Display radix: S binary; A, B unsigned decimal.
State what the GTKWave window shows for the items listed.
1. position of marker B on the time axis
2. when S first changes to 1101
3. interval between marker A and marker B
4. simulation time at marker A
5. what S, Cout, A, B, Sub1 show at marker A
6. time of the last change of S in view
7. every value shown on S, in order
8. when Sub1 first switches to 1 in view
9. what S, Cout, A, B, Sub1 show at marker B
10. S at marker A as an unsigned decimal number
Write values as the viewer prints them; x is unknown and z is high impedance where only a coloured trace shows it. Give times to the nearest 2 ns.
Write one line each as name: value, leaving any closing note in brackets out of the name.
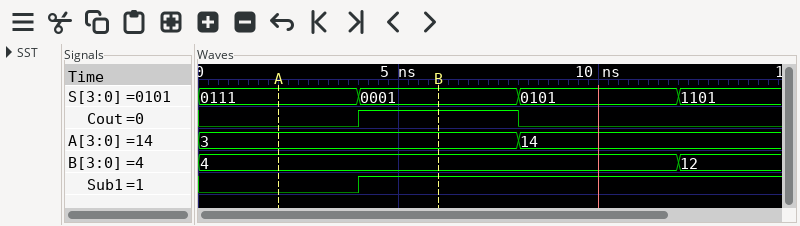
position of marker B on the time axis: 6 ns
when S first changes to 1101: 12 ns
interval between marker A and marker B: 4 ns
simulation time at marker A: 2 ns
what S, Cout, A, B, Sub1 show at marker A: S=0111, Cout=0, A=3, B=4, Sub1=0
time of the last change of S in view: 12 ns
every value shown on S, in order: 0111, 0001, 0101, 1101
when Sub1 first switches to 1 in view: 4 ns
what S, Cout, A, B, Sub1 show at marker B: S=0001, Cout=1, A=3, B=4, Sub1=1
S at marker A as an unsigned decimal number: 7
